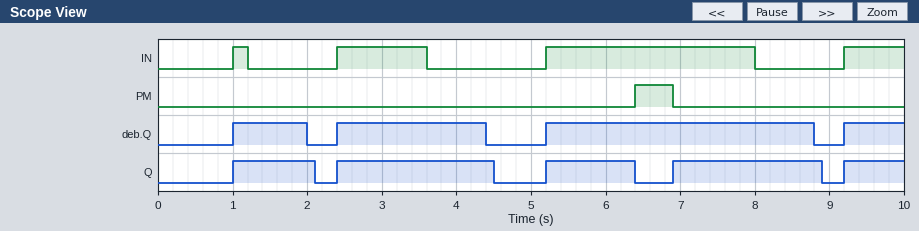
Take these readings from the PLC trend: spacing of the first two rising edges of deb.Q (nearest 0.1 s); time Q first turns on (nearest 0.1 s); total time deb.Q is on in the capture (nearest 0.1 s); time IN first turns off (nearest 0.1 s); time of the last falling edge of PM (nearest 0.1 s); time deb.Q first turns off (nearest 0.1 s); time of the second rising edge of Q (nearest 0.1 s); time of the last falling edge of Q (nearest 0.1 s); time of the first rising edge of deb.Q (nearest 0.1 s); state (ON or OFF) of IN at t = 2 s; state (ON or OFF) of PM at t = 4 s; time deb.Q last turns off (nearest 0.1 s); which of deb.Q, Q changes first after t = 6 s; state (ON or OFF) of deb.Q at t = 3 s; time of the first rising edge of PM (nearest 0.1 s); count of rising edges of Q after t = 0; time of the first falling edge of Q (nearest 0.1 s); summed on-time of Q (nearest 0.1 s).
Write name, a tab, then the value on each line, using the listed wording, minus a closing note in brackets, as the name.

spacing of the first two rising edges of deb.Q	1.4 s
time Q first turns on	1.0 s
total time deb.Q is on in the capture	7.4 s
time IN first turns off	1.2 s
time of the last falling edge of PM	6.9 s
time deb.Q first turns off	2.0 s
time of the second rising edge of Q	2.4 s
time of the last falling edge of Q	8.9 s
time of the first rising edge of deb.Q	1.0 s
state (ON or OFF) of IN at t = 2 s	OFF
state (ON or OFF) of PM at t = 4 s	OFF
time deb.Q last turns off	8.8 s
which of deb.Q, Q changes first after t = 6 s	Q
state (ON or OFF) of deb.Q at t = 3 s	ON
time of the first rising edge of PM	6.4 s
count of rising edges of Q after t = 0	5
time of the first falling edge of Q	2.1 s
summed on-time of Q	7.2 s
